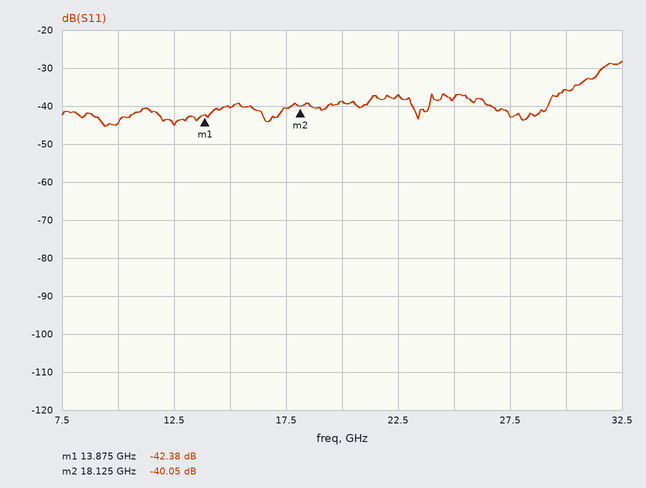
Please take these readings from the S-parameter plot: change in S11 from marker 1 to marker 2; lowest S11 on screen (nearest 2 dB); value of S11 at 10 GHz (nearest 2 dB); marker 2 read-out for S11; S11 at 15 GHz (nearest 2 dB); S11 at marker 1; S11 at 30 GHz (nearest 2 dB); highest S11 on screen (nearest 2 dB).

2.33 dB
-46 dB
-44 dB
-40.05 dB
-40 dB
-42.38 dB
-36 dB
-28 dB
